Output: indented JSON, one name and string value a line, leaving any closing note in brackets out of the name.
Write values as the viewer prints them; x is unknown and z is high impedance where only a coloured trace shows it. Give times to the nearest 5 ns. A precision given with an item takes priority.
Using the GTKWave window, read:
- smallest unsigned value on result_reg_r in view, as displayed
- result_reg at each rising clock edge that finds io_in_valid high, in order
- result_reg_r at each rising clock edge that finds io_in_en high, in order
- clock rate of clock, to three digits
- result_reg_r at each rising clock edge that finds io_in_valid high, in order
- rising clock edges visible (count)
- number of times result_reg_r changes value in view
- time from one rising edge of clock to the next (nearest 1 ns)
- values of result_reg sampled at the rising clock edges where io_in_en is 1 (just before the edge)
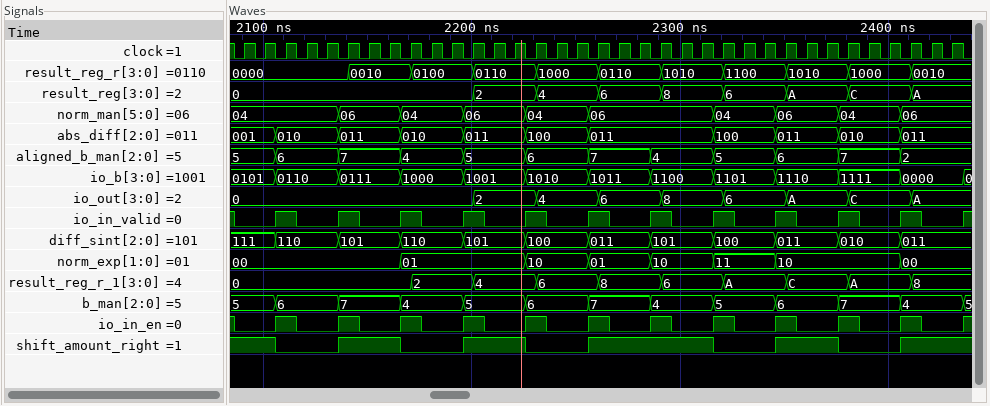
{
  "smallest unsigned value on result_reg_r in view, as displayed": "0000",
  "result_reg at each rising clock edge that finds io_in_valid high, in order": "0, 0, 0, 0, 2, 4, 6, 8, 6, A, C",
  "result_reg_r at each rising clock edge that finds io_in_en high, in order": "0000, 0000, 0010, 0100, 0110, 1000, 0110, 1010, 1100, 1010, 1000",
  "clock rate of clock, to three digits": "100 MHz",
  "result_reg_r at each rising clock edge that finds io_in_valid high, in order": "0000, 0000, 0010, 0100, 0110, 1000, 0110, 1010, 1100, 1010, 1000",
  "rising clock edges visible": "35",
  "number of times result_reg_r changes value in view": "10",
  "time from one rising edge of clock to the next": "10 ns",
  "values of result_reg sampled at the rising clock edges where io_in_en is 1": "0, 0, 0, 0, 2, 4, 6, 8, 6, A, C"
}
